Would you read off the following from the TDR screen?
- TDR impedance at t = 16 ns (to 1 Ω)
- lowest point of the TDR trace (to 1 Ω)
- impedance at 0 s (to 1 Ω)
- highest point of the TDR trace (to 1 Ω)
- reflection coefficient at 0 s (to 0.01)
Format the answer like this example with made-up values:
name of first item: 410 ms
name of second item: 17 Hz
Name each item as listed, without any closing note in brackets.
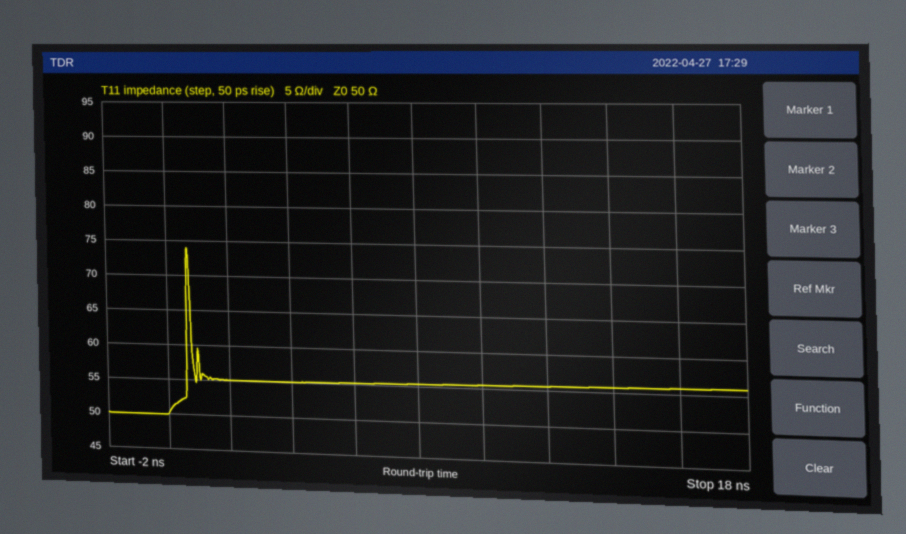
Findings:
TDR impedance at t = 16 ns: 56 Ω
lowest point of the TDR trace: 50 Ω
impedance at 0 s: 50 Ω
highest point of the TDR trace: 74 Ω
reflection coefficient at 0 s: 0.00
